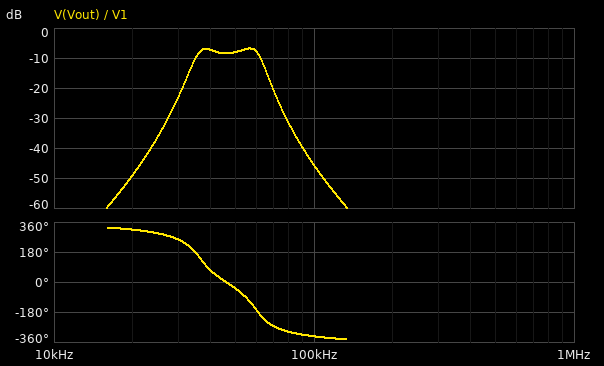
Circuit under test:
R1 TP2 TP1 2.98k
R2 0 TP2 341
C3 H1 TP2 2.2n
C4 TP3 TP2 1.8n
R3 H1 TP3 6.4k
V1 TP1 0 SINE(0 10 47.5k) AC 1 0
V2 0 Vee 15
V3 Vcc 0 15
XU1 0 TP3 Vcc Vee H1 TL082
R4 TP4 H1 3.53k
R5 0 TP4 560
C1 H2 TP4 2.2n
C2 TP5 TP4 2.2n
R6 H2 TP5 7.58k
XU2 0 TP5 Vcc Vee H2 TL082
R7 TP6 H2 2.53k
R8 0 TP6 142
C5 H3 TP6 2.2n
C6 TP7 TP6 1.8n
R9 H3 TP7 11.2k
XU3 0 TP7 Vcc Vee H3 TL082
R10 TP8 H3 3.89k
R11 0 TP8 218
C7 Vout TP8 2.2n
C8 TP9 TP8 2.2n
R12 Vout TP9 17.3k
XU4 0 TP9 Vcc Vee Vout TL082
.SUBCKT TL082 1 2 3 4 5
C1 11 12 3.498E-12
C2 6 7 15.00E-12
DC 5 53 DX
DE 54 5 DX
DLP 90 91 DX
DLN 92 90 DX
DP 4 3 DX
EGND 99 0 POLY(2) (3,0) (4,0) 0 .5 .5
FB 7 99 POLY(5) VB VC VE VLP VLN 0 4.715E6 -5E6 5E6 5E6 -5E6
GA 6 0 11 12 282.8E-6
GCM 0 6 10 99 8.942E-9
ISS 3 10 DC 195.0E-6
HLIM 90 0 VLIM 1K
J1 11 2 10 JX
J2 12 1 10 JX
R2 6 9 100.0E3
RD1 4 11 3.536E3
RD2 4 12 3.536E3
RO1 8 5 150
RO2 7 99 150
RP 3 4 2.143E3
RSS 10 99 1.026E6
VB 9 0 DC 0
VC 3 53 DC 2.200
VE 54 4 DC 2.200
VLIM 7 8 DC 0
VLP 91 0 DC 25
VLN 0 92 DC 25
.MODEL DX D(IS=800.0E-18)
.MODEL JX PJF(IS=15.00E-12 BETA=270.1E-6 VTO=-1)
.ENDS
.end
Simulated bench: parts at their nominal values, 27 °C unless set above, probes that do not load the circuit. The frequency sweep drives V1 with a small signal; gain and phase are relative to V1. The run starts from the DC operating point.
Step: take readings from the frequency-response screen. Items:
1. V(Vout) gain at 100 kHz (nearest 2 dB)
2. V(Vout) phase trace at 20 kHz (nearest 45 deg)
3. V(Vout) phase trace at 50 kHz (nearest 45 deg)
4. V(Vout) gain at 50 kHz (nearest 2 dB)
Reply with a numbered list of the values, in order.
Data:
1. -46 dB
2. 315 deg
3. -45 deg
4. -8 dB
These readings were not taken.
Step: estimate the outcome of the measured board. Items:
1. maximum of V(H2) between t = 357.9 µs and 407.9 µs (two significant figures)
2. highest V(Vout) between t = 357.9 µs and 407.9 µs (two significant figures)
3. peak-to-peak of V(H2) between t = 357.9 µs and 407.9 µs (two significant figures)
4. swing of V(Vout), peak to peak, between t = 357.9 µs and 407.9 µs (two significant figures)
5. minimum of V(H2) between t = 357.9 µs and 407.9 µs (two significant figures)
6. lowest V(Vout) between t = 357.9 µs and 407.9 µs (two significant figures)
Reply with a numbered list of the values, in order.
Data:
1. 6.0 V
2. 3.8 V
3. 12 V
4. 7.6 V
5. -6.0 V
6. -3.8 V
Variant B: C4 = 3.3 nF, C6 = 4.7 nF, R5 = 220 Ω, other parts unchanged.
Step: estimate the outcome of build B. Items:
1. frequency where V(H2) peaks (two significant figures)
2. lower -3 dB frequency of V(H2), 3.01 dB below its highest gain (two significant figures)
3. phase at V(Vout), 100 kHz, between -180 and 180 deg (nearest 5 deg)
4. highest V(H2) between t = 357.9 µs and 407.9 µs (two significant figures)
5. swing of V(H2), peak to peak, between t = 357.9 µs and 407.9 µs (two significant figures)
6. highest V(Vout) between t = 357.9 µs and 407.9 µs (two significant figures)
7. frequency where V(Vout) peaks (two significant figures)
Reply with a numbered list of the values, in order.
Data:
1. 51 kHz
2. 40 kHz
3. 25 deg
4. 8.5 V
5. 17 V
6. 8.7 V
7. 38 kHz
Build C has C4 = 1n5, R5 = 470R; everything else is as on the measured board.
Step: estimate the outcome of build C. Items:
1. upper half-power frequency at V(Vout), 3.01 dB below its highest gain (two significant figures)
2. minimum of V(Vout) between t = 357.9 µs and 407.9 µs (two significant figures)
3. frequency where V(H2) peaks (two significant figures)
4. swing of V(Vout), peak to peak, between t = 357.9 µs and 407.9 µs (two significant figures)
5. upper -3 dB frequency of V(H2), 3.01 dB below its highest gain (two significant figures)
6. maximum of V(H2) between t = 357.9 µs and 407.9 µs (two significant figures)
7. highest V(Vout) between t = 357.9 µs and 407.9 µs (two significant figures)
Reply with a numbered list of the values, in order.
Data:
1. 63 kHz
2. -3.1 V
3. 52 kHz
4. 6.3 V
5. 66 kHz
6. 4.9 V
7. 3.1 V
